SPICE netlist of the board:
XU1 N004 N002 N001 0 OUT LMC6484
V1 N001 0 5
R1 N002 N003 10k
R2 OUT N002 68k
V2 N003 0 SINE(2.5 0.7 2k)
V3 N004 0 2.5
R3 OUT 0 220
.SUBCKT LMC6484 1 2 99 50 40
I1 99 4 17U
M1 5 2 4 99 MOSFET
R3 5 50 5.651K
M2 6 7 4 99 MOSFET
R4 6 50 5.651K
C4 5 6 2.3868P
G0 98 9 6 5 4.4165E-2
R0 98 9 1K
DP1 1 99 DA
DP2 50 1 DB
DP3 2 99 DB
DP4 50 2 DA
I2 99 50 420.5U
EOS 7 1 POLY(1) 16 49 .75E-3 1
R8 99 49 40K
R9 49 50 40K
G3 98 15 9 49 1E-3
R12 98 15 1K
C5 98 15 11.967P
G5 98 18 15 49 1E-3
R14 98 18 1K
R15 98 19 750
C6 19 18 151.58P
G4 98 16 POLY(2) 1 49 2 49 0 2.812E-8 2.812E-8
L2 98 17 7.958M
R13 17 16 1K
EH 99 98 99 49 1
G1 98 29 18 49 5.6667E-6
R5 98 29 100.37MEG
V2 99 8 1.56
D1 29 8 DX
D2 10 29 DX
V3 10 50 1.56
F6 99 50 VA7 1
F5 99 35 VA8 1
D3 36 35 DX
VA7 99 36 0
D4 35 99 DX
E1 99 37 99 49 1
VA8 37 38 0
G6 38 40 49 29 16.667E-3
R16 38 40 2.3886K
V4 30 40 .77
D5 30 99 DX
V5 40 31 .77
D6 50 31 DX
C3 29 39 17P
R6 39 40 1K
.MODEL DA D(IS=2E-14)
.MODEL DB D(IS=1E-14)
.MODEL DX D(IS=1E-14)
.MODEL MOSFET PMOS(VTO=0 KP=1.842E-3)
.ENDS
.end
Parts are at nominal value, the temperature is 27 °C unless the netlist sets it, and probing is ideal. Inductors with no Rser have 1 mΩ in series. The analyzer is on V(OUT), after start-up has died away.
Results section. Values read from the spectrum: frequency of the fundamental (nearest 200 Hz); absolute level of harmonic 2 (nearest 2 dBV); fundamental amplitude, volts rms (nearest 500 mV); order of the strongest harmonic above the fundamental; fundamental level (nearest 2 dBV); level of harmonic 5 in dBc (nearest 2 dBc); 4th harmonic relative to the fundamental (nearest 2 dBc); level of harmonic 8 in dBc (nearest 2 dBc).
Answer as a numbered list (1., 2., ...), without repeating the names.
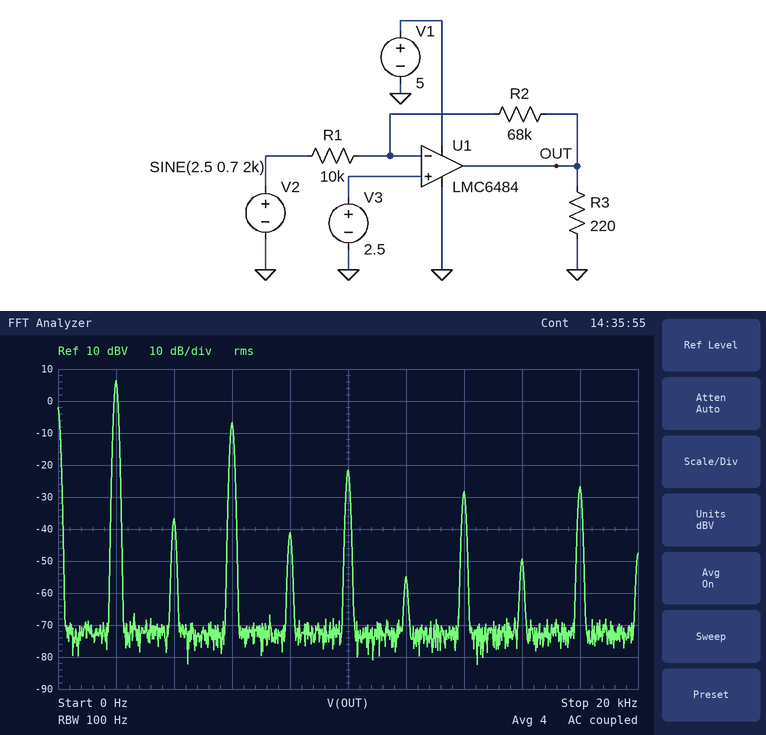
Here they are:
1. 2.0 kHz
2. -36 dBV
3. 2.0 V
4. 3
5. 6 dBV
6. -28 dBc
7. -48 dBc
8. -56 dBc
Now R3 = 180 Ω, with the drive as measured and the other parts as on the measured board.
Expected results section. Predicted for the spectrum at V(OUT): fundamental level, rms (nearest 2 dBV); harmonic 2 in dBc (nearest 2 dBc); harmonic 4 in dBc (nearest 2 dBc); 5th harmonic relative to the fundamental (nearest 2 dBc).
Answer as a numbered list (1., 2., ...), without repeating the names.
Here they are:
1. 6 dBV
2. -24 dBc
3. -28 dBc
4. -24 dBc
